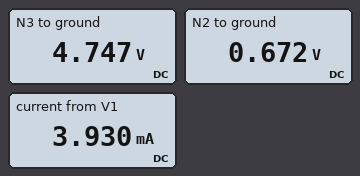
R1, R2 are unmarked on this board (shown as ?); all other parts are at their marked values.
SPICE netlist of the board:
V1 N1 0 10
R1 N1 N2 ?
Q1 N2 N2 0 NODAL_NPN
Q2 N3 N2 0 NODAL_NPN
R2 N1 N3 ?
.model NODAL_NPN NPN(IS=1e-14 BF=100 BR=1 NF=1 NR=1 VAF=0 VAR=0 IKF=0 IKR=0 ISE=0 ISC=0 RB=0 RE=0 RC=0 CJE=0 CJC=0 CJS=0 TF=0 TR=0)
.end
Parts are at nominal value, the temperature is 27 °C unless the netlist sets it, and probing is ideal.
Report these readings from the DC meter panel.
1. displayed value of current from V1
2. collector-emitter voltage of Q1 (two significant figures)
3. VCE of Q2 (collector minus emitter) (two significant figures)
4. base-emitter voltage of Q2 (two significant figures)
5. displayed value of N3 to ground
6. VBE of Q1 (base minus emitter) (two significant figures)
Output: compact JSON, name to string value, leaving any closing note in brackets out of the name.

{"displayed value of current from V1": "3.930 mA", "collector-emitter voltage of Q1": "670 mV", "VCE of Q2 (collector minus emitter)": "4.7 V", "base-emitter voltage of Q2": "670 mV", "displayed value of N3 to ground": "4.747 V", "VBE of Q1 (base minus emitter)": "670 mV"}
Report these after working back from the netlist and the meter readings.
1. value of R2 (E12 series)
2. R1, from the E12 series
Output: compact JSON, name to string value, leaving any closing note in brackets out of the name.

{"value of R2": "2.7 kΩ", "R1, from the E12 series": "4.7 kΩ"}
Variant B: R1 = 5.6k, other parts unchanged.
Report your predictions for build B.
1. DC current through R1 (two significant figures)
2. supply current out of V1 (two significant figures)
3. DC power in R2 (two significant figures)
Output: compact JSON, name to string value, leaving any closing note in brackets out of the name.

{"DC current through R1": "1.7 mA", "supply current out of V1": "3.3 mA", "DC power in R2": "7.2 mW"}
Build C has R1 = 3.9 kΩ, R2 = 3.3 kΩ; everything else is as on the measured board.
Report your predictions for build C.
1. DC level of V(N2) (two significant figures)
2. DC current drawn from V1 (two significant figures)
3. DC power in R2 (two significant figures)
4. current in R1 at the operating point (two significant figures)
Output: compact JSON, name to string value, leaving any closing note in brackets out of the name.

{"DC level of V(N2)": "680 mV", "DC current drawn from V1": "4.7 mA", "DC power in R2": "18 mW", "current in R1 at the operating point": "2.4 mA"}
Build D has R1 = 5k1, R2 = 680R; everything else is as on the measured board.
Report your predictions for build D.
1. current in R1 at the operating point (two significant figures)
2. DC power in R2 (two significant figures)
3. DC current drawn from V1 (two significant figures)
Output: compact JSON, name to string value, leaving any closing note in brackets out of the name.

{"current in R1 at the operating point": "1.8 mA", "DC power in R2": "2.2 mW", "DC current drawn from V1": "3.6 mA"}
